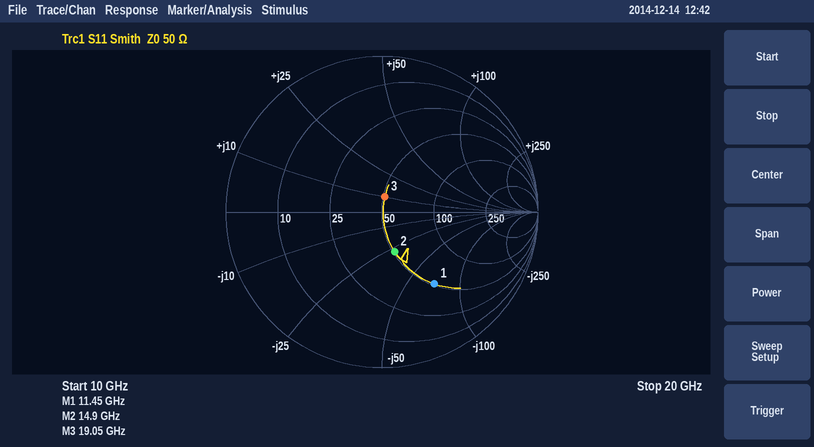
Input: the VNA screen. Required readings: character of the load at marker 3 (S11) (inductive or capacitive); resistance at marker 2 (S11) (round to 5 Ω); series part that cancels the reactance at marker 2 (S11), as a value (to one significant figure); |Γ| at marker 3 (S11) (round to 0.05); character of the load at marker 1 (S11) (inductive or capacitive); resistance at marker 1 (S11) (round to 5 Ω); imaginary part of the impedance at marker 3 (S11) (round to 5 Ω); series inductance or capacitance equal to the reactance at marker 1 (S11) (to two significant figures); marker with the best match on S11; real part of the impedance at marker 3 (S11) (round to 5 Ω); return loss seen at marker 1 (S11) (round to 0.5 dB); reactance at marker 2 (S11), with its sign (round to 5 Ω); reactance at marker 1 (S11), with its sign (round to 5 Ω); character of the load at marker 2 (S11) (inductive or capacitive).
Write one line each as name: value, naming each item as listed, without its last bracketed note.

character of the load at marker 3 (S11): inductive
resistance at marker 2 (S11): 50 Ω
series part that cancels the reactance at marker 2 (S11), as a value: 300 pH
|Γ| at marker 3 (S11): 0.10
character of the load at marker 1 (S11): capacitive
resistance at marker 1 (S11): 50 Ω
imaginary part of the impedance at marker 3 (S11): +10 Ω
series inductance or capacitance equal to the reactance at marker 1 (S11): 200 fF
marker with the best match on S11: marker 3
real part of the impedance at marker 3 (S11): 50 Ω
return loss seen at marker 1 (S11): 5.0 dB
reactance at marker 2 (S11), with its sign: -30 Ω
reactance at marker 1 (S11), with its sign: -70 Ω
character of the load at marker 2 (S11): capacitive
